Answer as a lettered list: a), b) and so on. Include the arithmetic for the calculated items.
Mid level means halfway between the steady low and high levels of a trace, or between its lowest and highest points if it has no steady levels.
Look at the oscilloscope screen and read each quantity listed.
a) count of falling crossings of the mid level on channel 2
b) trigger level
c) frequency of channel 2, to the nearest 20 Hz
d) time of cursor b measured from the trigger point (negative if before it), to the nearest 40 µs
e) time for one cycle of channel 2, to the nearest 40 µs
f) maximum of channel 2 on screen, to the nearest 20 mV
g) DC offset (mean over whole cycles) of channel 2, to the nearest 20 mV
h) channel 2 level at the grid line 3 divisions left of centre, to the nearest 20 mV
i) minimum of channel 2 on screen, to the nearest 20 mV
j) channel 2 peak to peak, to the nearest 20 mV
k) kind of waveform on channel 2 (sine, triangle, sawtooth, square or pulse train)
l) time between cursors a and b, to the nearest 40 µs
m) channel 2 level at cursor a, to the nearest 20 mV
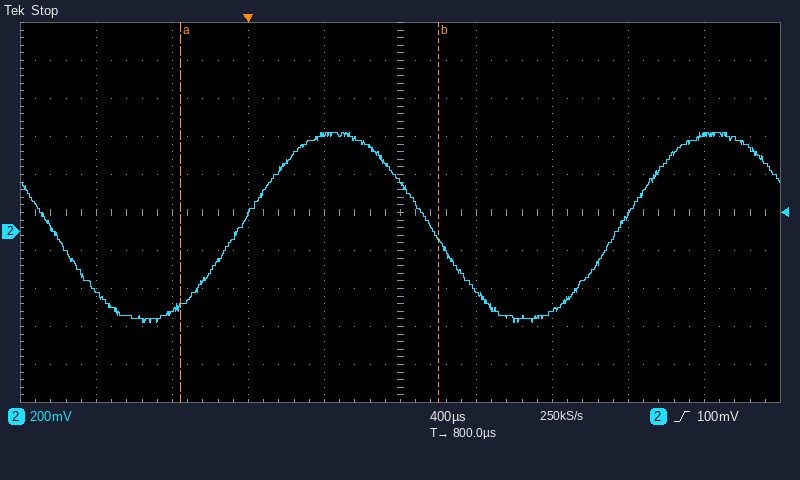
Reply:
a) 2
b) 100 mV
c) 1 / 2.00 ms ≈ 500 Hz
d) +1.00 ms
e) 2.00 ms
f) 520 mV
g) (520 mV + (-480 mV)) / 2 ≈ 20 mV
h) -420 mV
i) -480 mV
j) 520 mV − (-480 mV) = 1.00 V
k) sine
l) 1.36 ms
m) -400 mV
